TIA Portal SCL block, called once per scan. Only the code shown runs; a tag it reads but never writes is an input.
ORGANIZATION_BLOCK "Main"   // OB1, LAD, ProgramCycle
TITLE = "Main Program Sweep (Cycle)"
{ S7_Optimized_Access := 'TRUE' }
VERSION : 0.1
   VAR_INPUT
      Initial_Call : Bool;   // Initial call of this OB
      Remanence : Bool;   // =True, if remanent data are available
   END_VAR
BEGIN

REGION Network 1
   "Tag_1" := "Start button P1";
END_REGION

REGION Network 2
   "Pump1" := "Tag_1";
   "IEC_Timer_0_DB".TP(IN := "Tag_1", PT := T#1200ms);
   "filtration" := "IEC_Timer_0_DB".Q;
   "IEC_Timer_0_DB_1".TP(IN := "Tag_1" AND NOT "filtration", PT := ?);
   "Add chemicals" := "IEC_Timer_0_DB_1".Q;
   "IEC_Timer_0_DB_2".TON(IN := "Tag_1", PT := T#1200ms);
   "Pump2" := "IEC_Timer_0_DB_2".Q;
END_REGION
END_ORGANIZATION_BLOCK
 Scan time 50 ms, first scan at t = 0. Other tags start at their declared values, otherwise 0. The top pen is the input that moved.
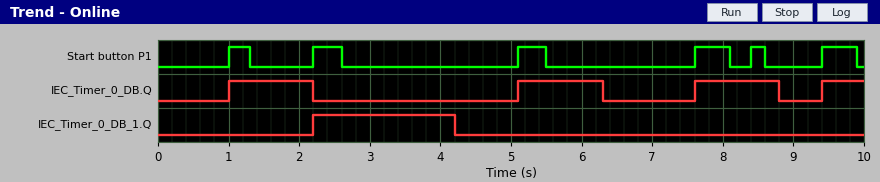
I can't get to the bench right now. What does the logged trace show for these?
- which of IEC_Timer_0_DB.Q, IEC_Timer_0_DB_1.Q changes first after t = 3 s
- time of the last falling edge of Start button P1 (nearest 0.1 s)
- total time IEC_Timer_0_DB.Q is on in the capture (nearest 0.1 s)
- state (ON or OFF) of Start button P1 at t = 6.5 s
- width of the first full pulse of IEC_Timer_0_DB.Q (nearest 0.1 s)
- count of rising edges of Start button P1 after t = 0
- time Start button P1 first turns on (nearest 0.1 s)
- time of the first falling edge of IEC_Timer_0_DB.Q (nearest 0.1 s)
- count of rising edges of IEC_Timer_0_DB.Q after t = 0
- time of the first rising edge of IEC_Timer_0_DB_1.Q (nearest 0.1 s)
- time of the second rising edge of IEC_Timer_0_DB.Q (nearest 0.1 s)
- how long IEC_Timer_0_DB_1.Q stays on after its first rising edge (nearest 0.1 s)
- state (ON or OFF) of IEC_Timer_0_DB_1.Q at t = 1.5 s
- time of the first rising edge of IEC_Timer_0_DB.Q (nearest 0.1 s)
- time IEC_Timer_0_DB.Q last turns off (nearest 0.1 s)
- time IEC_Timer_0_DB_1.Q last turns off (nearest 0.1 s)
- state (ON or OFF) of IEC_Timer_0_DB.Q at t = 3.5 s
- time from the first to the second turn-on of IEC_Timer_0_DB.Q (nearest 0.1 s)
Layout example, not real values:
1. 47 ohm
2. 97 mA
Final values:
1. IEC_Timer_0_DB_1.Q
2. 9.9 s
3. 4.2 s
4. OFF
5. 1.2 s
6. 6
7. 1.0 s
8. 2.2 s
9. 4
10. 2.2 s
11. 5.1 s
12. 2.0 s
13. OFF
14. 1.0 s
15. 8.8 s
16. 4.2 s
17. OFF
18. 4.1 s
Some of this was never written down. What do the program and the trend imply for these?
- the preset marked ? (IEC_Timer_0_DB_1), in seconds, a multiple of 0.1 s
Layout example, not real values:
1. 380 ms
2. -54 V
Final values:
1. 2.0 s
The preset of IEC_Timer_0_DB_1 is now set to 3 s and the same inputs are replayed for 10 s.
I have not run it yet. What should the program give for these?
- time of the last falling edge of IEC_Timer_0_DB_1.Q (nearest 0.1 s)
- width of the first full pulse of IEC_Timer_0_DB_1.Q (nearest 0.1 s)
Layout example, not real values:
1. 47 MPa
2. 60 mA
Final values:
1. 5.2 s
2. 3.0 s
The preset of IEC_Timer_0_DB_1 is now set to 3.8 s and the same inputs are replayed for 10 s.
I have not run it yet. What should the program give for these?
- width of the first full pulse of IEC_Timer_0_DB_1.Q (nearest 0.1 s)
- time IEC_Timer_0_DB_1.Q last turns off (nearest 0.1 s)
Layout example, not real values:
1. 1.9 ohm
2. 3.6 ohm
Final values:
1. 3.8 s
2. 6.0 s
